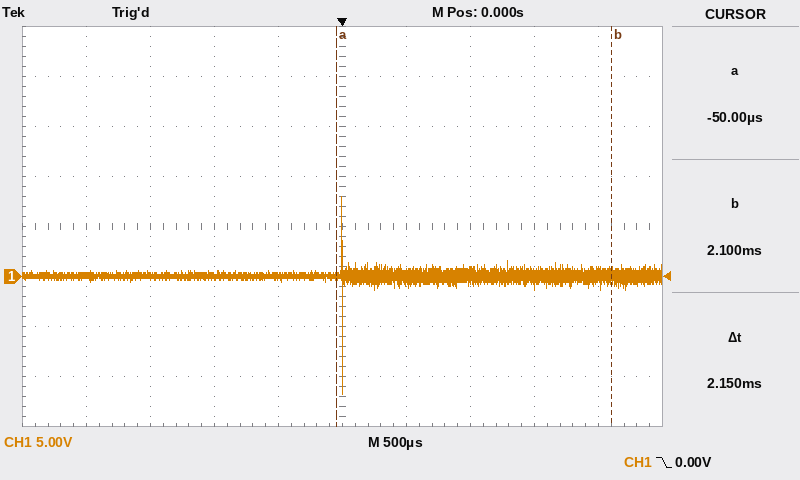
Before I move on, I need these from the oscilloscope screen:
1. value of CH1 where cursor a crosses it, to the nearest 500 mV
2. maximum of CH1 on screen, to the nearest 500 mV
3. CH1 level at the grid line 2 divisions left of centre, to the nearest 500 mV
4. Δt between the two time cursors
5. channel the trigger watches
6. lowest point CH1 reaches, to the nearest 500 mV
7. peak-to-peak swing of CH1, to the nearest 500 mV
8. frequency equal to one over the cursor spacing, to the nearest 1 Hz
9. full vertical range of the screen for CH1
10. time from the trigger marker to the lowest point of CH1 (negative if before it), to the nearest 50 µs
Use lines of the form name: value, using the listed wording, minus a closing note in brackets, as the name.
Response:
value of CH1 where cursor a crosses it, to the nearest 500 mV: 0.0 V
maximum of CH1 on screen, to the nearest 500 mV: 8.0 V
CH1 level at the grid line 2 divisions left of centre, to the nearest 500 mV: 0.0 V
Δt between the two time cursors: 2.15 ms
channel the trigger watches: CH1
lowest point CH1 reaches, to the nearest 500 mV: -12.0 V
peak-to-peak swing of CH1, to the nearest 500 mV: 20.0 V
frequency equal to one over the cursor spacing, to the nearest 1 Hz: 465 Hz
full vertical range of the screen for CH1: 40 V
time from the trigger marker to the lowest point of CH1 (negative if before it), to the nearest 50 µs: 0 µs
